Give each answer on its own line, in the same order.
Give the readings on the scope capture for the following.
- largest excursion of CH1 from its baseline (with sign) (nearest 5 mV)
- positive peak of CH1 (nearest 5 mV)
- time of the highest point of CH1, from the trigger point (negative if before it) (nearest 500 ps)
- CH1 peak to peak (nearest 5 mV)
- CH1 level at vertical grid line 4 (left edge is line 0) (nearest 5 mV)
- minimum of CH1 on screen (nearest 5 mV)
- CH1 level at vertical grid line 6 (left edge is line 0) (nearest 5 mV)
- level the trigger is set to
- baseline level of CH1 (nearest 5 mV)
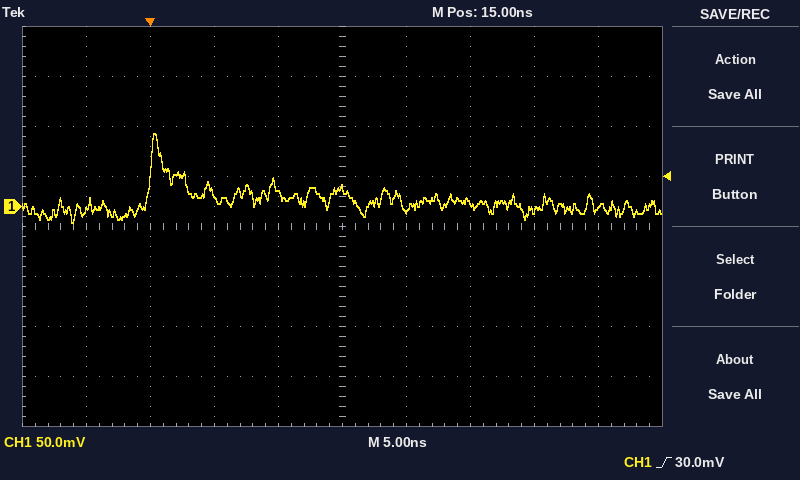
+70 mV
75 mV
+500 ps
90 mV
15 mV
-15 mV
-5 mV
30.0 mV
5 mV
